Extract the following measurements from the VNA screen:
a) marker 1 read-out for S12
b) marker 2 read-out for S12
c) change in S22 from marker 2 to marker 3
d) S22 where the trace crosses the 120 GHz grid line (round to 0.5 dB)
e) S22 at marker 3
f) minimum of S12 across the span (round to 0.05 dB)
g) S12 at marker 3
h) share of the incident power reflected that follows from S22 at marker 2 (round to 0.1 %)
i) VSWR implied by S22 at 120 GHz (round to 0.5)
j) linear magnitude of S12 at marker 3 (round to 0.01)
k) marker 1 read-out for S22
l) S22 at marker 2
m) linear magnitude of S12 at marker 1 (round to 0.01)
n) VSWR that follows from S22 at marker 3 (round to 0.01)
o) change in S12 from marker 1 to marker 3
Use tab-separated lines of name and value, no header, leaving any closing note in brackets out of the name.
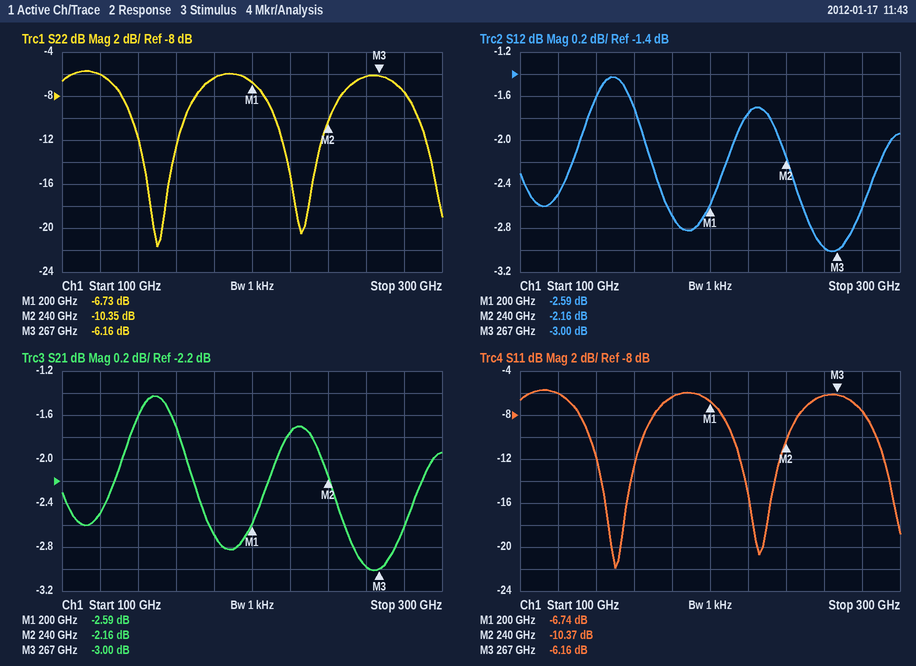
marker 1 read-out for S12	-2.59 dB
marker 2 read-out for S12	-2.16 dB
change in S22 from marker 2 to marker 3	4.19 dB
S22 where the trace crosses the 120 GHz grid line	-6.0 dB
S22 at marker 3	-6.16 dB
minimum of S12 across the span	-3.00 dB
S12 at marker 3	-3.00 dB
share of the incident power reflected that follows from S22 at marker 2	9.2 %
VSWR implied by S22 at 120 GHz	3.0
linear magnitude of S12 at marker 3	0.71
marker 1 read-out for S22	-6.73 dB
S22 at marker 2	-10.35 dB
linear magnitude of S12 at marker 1	0.74
VSWR that follows from S22 at marker 3	2.94
change in S12 from marker 1 to marker 3	-0.41 dB
